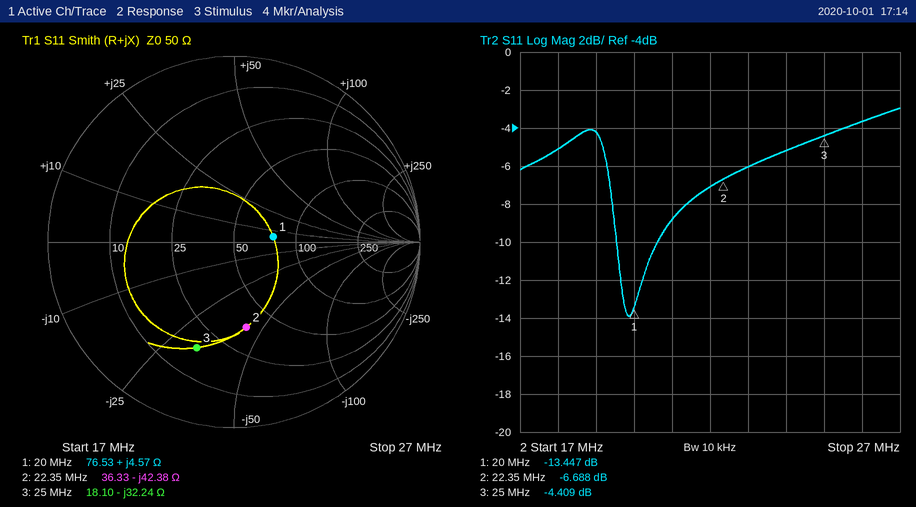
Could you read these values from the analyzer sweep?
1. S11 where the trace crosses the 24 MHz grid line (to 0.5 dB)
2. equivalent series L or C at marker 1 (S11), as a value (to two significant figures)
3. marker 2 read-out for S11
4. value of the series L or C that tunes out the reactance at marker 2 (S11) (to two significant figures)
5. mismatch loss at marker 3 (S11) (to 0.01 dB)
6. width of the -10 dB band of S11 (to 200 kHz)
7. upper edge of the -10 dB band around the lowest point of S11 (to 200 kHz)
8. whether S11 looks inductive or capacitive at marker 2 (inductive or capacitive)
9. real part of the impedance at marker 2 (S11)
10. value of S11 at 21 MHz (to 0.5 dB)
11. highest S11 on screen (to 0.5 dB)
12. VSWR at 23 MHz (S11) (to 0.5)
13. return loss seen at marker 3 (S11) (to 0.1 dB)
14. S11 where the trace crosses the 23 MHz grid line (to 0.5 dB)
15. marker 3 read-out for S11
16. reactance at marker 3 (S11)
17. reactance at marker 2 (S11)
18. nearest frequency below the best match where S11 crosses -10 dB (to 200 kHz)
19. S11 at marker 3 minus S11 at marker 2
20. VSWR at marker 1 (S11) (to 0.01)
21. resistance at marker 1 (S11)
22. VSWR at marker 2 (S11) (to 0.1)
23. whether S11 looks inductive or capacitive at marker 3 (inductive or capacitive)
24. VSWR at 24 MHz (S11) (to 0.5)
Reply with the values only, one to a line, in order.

-5.0 dB
36 nH
-6.688 dB
300 nH
1.95 dB
1.0 MHz
20.6 MHz
capacitive
36.33 Ω
-9.0 dB
-3.0 dB
3.0
4.4 dB
-6.0 dB
-4.409 dB
-32.24 Ω
-42.38 Ω
19.6 MHz
2.279 dB
1.54
76.53 Ω
2.7
capacitive
3.5
